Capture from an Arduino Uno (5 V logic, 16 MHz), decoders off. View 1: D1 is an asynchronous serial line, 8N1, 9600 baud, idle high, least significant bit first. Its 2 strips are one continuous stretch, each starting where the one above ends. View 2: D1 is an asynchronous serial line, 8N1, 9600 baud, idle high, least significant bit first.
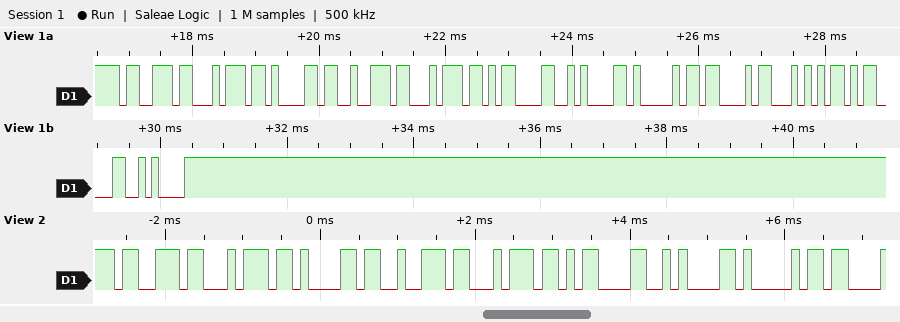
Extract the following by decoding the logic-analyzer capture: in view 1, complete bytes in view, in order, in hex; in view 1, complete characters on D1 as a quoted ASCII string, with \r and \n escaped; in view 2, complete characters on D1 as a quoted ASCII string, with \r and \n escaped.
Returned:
0x73 0x74 0x61 0x72 0x74 0x0D 0x0A 0x41 0x43 0x54 0x0D 0x0A
"start\r\nACT\r\n"
"start\r\nA"
